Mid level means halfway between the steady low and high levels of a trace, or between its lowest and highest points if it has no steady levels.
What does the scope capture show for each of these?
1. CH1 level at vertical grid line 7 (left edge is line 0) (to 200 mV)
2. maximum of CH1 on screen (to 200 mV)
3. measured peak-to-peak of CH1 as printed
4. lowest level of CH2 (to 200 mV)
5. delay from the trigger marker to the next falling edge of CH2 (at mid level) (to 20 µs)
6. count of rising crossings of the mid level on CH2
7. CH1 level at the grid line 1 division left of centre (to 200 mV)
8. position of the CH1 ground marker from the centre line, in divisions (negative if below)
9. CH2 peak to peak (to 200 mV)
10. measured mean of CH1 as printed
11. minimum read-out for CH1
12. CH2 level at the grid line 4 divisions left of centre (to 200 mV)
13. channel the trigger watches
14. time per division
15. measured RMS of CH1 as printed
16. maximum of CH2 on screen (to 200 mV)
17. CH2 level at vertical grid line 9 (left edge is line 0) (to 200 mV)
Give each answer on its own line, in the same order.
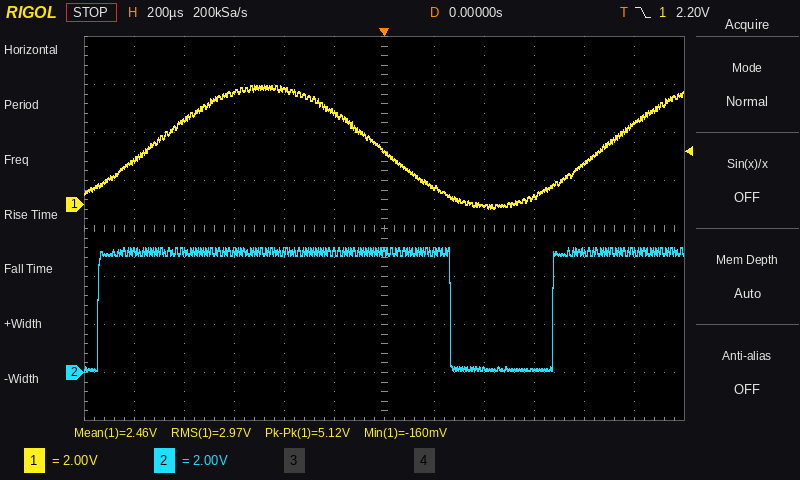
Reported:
800 mV
5.0 V
5.12 V
0.0 V
260 µs
2
3.8 V
+0.5 div
5.2 V
2.46 V
-160 mV
5.0 V
CH1
200 µs
2.97 V
5.2 V
200 mV
